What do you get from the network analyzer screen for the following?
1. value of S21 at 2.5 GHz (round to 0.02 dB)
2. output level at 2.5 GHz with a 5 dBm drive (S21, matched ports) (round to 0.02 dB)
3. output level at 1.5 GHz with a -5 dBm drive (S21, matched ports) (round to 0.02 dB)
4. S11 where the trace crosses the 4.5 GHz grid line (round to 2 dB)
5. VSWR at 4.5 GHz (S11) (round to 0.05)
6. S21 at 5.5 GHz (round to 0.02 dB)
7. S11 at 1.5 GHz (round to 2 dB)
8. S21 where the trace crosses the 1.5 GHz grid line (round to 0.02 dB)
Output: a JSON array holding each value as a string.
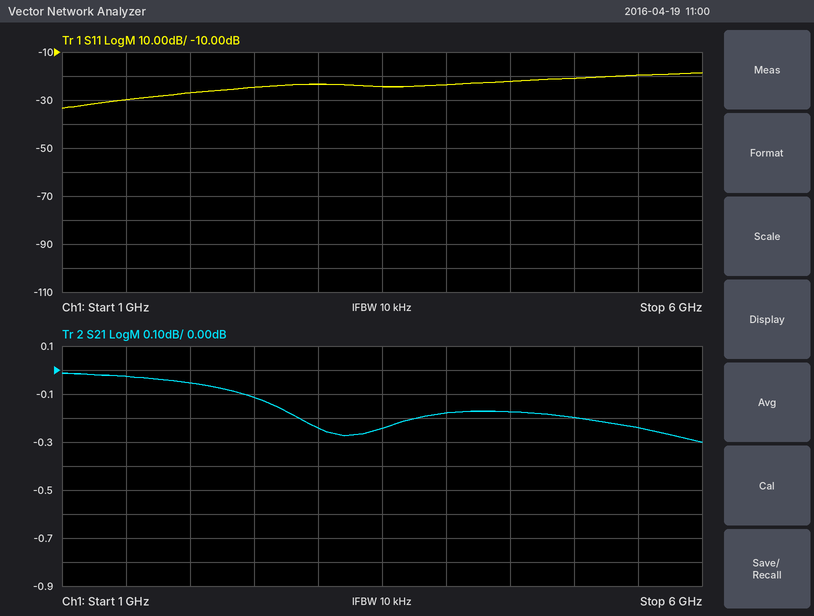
["-0.12 dB", "4.88 dBm", "-5.02 dBm", "-22 dB", "1.15", "-0.24 dB", "-30 dB", "-0.02 dB"]
